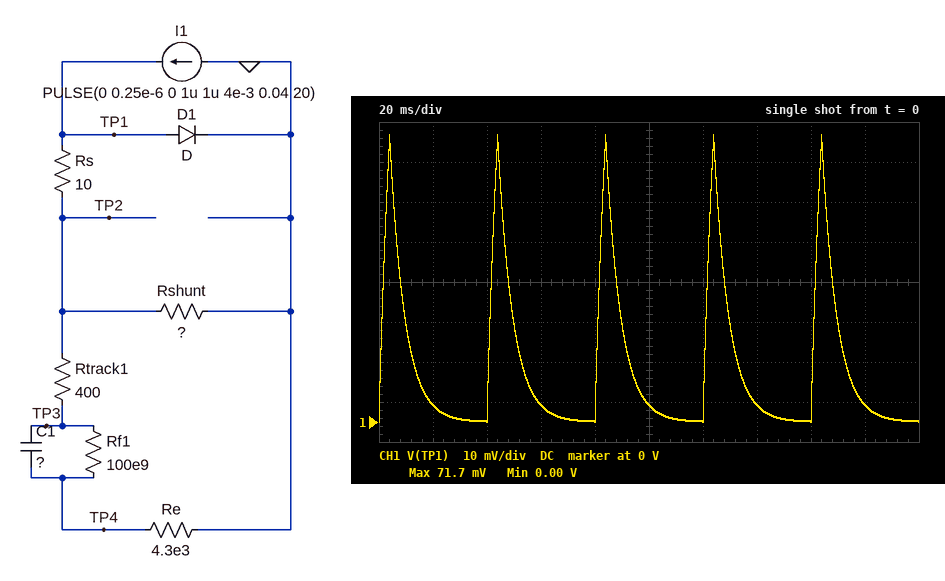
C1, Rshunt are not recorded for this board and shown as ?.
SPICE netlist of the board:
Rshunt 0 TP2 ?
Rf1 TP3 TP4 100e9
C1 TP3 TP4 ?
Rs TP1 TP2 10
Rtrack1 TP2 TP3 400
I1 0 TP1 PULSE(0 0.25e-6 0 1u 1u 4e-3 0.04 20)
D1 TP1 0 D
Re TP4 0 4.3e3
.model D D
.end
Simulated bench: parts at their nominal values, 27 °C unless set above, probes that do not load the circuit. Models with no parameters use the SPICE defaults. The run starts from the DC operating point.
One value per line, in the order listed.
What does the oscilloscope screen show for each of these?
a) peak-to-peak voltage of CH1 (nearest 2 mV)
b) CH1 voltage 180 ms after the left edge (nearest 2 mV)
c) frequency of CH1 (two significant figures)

72 mV
4 mV
25 Hz
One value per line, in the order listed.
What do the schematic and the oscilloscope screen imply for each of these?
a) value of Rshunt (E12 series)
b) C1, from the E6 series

560 kΩ
10 nF
